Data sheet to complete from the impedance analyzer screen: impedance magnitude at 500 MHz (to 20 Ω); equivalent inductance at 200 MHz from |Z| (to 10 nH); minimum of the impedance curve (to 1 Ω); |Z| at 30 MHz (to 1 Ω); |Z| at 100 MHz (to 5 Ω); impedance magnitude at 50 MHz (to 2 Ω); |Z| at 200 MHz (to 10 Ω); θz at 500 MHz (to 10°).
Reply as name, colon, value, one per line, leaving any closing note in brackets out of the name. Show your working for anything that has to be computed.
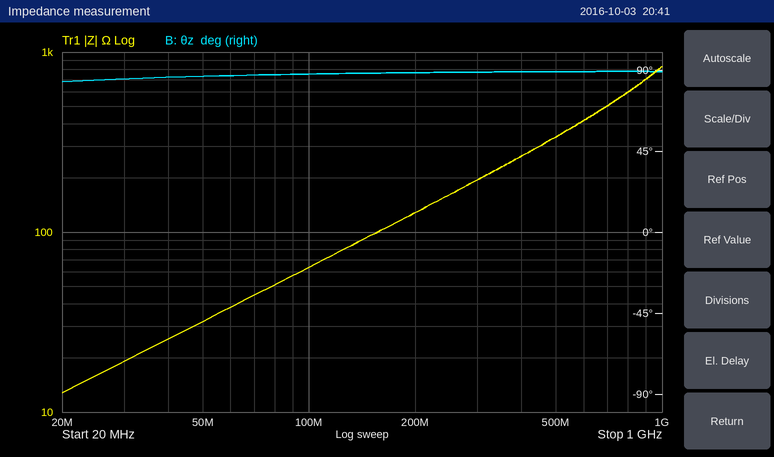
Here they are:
impedance magnitude at 500 MHz: 340 Ω
equivalent inductance at 200 MHz from |Z|: L = 130 Ω/(2π × 200 MHz) ≈ 103 nH, so 100 nH to the nearest 10 nH
minimum of the impedance curve: 13 Ω
|Z| at 30 MHz: 19 Ω
|Z| at 100 MHz: 65 Ω
impedance magnitude at 50 MHz: 32 Ω
|Z| at 200 MHz: 130 Ω
θz at 500 MHz: 90°
